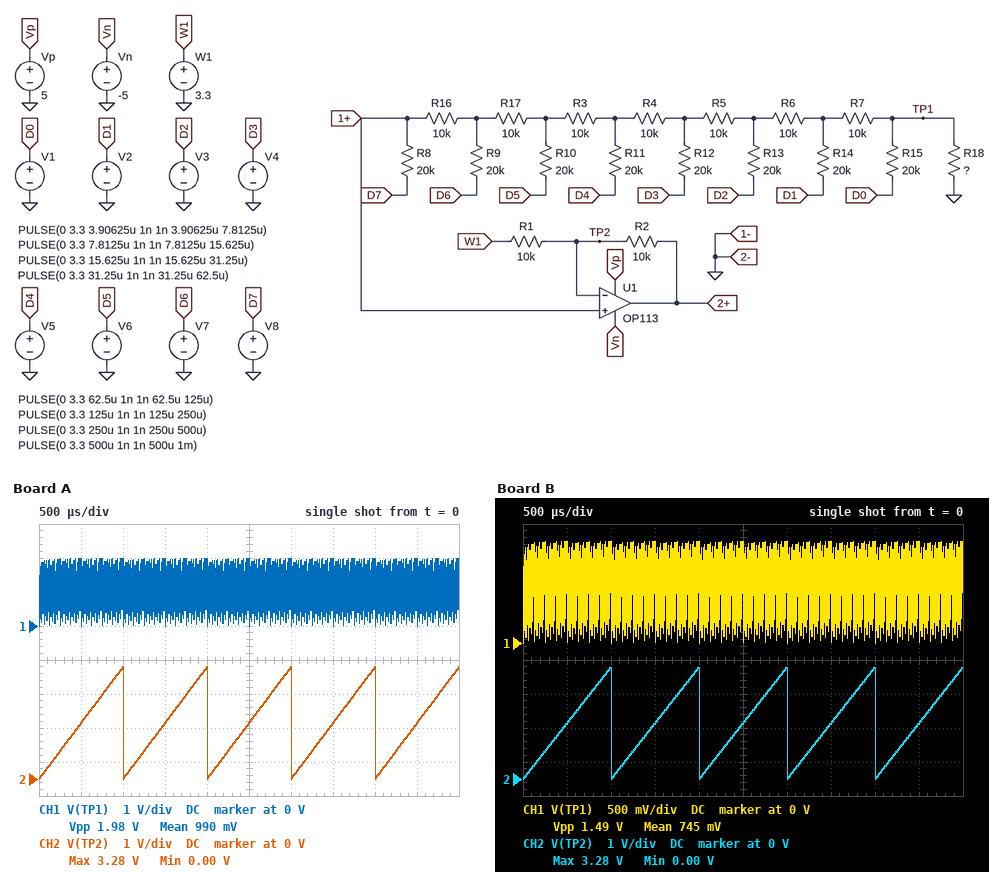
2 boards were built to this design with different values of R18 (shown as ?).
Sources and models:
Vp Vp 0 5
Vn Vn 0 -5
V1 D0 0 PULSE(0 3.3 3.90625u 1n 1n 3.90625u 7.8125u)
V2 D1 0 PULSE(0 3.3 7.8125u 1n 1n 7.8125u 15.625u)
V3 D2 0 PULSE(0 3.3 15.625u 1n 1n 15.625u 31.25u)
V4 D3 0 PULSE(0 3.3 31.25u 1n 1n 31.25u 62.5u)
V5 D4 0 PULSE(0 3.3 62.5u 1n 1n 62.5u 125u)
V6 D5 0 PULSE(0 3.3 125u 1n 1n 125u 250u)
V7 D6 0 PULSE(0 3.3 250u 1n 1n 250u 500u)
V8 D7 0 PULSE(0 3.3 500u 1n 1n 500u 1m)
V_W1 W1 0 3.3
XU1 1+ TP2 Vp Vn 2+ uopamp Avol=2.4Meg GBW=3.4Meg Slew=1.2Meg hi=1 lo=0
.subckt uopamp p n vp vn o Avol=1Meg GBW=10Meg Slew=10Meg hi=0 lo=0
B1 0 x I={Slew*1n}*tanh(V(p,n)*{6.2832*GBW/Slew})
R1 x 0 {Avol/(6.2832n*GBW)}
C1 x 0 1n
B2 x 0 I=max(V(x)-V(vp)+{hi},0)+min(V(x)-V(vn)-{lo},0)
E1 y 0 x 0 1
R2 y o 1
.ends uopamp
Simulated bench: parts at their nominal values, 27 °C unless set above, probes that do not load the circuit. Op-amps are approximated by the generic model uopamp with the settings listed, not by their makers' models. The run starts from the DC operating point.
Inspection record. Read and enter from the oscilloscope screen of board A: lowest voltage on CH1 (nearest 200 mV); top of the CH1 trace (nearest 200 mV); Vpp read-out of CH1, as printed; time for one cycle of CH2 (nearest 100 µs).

0 V
2.0 V
1.98 V
1.0 ms
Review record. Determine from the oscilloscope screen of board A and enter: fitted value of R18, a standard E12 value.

15 kΩ
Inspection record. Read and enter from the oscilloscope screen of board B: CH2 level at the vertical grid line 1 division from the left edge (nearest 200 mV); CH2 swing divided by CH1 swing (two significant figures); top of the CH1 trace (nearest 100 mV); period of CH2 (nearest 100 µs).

1.6 V
2.2
1.5 V
1.0 ms
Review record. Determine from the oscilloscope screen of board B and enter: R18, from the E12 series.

8.2 kΩ
